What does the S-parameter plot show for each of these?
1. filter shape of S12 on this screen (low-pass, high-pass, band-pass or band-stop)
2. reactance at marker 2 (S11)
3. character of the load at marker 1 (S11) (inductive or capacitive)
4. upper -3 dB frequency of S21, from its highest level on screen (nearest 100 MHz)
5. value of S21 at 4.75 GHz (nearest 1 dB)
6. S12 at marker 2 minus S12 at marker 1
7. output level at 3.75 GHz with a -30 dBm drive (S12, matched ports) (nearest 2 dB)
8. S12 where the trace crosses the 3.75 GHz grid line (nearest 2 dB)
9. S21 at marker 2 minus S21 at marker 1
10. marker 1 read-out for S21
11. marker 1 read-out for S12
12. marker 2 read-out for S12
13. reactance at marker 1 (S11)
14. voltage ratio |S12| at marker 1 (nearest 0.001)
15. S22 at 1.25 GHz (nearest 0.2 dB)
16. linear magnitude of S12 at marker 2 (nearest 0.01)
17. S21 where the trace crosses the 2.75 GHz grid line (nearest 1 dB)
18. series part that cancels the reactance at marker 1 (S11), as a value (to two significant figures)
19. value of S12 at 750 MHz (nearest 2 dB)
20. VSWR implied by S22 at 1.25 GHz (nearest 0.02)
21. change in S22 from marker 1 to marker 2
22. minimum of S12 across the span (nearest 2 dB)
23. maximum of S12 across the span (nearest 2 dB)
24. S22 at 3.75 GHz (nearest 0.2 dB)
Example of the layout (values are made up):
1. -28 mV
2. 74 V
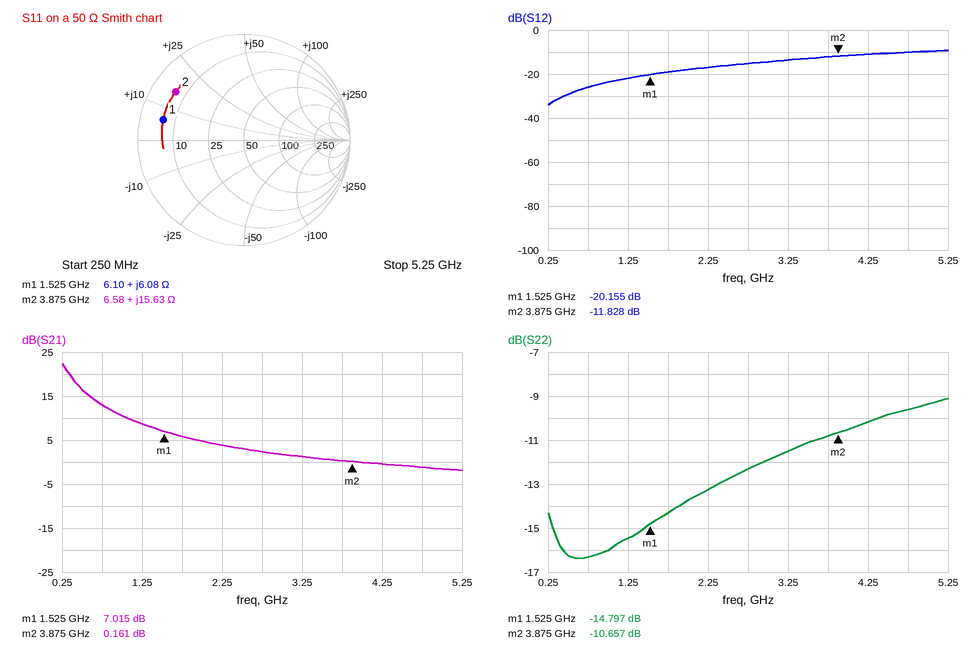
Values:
1. high-pass
2. +15.63 Ω
3. inductive
4. 400 MHz
5. -1 dB
6. 8.327 dB
7. -42 dBm
8. -12 dB
9. -6.854 dB
10. 7.015 dB
11. -20.155 dB
12. -11.828 dB
13. +6.08 Ω
14. 0.098
15. -15.4 dB
16. 0.26
17. 2 dB
18. 17 pF
19. -26 dB
20. 1.40
21. 4.140 dB
22. -34 dB
23. -10 dB
24. -10.8 dB
